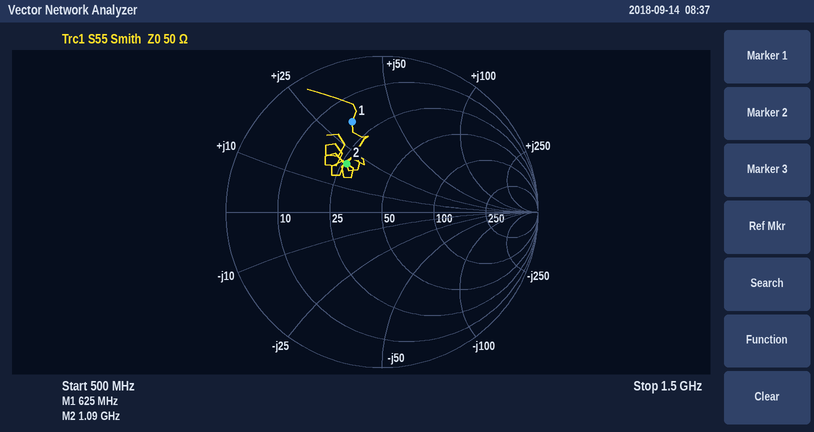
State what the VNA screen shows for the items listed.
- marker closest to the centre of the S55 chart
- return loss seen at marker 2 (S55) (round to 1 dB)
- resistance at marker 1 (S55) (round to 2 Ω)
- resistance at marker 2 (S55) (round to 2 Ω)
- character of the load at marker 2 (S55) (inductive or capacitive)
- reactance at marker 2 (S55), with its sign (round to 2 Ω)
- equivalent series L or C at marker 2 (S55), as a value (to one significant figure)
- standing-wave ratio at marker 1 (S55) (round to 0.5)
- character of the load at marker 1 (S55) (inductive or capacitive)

marker 2
8 dB
18 Ω
26 Ω
inductive
+20 Ω
3 nH
4.0
inductive
